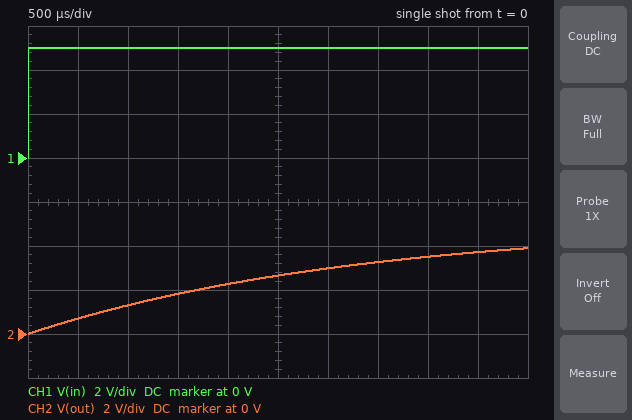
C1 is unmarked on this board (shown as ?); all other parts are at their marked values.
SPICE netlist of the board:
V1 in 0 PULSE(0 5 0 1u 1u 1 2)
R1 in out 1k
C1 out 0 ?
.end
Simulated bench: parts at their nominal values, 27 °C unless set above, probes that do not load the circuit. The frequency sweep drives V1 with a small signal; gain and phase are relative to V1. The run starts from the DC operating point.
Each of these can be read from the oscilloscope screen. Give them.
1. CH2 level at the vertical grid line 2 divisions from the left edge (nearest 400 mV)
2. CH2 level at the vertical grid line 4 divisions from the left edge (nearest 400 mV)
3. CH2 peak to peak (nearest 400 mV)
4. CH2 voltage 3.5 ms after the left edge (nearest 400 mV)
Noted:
1.2 V
2.4 V
4.0 V
3.2 V
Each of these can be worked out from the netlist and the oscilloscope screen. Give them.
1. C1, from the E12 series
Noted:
3.3 µF
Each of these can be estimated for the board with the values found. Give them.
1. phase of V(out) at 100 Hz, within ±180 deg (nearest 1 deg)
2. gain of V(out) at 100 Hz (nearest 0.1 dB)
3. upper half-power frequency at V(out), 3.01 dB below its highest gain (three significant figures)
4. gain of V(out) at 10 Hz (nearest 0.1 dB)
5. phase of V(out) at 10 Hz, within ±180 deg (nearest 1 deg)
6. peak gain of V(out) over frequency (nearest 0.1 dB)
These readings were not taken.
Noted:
-64 deg
-7.2 dB
48.2 Hz
-0.2 dB
-12 deg
0 dB
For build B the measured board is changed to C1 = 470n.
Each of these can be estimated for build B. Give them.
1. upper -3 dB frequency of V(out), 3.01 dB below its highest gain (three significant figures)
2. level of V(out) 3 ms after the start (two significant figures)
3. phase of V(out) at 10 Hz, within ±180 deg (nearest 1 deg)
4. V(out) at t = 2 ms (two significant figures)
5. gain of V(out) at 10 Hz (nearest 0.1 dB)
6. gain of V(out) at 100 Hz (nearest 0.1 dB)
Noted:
339 Hz
5.0 V
-2 deg
4.9 V
0 dB
-0.4 dB
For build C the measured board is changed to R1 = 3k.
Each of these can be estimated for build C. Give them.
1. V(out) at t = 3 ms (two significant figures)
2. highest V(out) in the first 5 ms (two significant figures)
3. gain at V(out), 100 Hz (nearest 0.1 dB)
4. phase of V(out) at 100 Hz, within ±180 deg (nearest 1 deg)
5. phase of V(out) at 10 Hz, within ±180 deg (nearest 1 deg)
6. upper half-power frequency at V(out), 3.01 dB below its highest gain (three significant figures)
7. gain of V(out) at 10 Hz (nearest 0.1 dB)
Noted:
1.3 V
2.0 V
-16.0 dB
-81 deg
-32 deg
16.1 Hz
-1.4 dB
